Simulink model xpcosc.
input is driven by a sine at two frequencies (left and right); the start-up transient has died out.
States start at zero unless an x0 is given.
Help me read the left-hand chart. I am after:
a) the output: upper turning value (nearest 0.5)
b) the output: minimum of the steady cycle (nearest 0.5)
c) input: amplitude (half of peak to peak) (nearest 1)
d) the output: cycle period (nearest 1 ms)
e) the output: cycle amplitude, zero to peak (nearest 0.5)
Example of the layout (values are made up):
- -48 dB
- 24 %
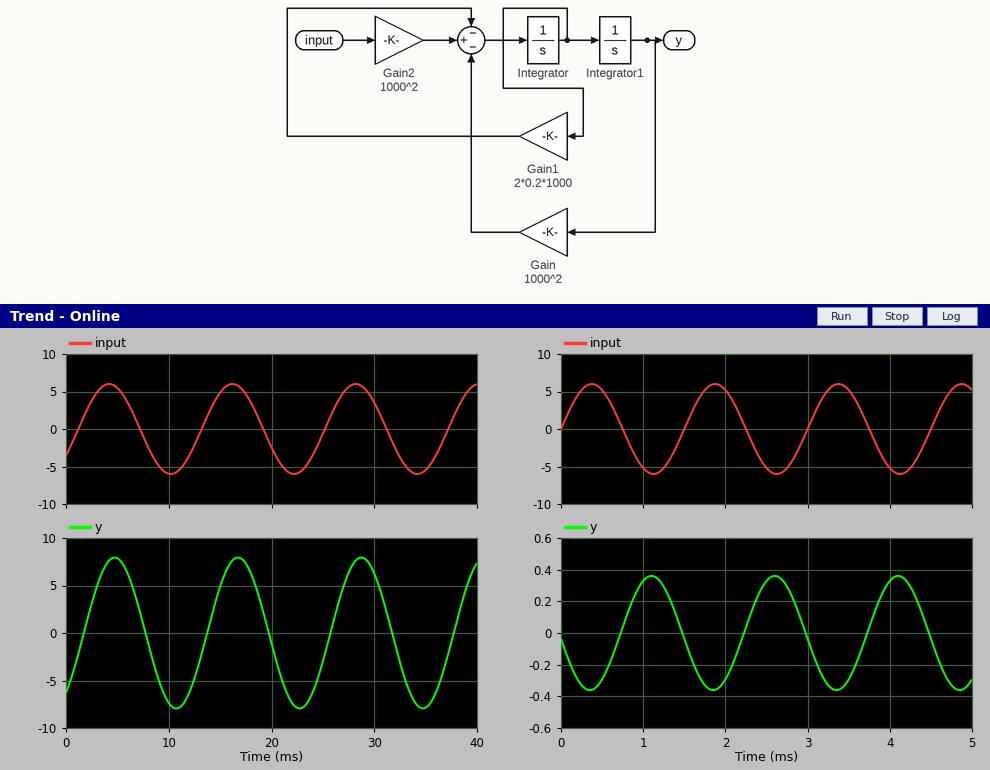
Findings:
- 8.0
- -8.0
- 6
- 12 ms
- 8.0
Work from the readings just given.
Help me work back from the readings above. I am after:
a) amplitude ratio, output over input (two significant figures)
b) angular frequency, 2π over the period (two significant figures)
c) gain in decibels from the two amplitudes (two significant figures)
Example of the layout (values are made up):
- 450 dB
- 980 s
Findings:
- 1.3
- 0.52 rad/ms
- 2.5 dB
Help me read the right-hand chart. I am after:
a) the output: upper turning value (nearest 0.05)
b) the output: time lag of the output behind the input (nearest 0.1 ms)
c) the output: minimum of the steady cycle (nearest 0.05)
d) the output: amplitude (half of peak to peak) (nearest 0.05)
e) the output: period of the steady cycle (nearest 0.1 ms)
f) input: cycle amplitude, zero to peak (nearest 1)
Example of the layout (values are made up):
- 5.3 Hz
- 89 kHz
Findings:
- 0.35
- 0.7 ms
- -0.35
- 0.35
- 1.5 ms
- 6
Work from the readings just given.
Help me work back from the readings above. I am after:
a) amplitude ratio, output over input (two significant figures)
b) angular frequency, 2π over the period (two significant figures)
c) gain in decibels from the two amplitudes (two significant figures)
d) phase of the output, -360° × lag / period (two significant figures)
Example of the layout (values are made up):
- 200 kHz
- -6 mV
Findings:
- 0.058
- 4.2 rad/ms
- -25 dB
- -170°
